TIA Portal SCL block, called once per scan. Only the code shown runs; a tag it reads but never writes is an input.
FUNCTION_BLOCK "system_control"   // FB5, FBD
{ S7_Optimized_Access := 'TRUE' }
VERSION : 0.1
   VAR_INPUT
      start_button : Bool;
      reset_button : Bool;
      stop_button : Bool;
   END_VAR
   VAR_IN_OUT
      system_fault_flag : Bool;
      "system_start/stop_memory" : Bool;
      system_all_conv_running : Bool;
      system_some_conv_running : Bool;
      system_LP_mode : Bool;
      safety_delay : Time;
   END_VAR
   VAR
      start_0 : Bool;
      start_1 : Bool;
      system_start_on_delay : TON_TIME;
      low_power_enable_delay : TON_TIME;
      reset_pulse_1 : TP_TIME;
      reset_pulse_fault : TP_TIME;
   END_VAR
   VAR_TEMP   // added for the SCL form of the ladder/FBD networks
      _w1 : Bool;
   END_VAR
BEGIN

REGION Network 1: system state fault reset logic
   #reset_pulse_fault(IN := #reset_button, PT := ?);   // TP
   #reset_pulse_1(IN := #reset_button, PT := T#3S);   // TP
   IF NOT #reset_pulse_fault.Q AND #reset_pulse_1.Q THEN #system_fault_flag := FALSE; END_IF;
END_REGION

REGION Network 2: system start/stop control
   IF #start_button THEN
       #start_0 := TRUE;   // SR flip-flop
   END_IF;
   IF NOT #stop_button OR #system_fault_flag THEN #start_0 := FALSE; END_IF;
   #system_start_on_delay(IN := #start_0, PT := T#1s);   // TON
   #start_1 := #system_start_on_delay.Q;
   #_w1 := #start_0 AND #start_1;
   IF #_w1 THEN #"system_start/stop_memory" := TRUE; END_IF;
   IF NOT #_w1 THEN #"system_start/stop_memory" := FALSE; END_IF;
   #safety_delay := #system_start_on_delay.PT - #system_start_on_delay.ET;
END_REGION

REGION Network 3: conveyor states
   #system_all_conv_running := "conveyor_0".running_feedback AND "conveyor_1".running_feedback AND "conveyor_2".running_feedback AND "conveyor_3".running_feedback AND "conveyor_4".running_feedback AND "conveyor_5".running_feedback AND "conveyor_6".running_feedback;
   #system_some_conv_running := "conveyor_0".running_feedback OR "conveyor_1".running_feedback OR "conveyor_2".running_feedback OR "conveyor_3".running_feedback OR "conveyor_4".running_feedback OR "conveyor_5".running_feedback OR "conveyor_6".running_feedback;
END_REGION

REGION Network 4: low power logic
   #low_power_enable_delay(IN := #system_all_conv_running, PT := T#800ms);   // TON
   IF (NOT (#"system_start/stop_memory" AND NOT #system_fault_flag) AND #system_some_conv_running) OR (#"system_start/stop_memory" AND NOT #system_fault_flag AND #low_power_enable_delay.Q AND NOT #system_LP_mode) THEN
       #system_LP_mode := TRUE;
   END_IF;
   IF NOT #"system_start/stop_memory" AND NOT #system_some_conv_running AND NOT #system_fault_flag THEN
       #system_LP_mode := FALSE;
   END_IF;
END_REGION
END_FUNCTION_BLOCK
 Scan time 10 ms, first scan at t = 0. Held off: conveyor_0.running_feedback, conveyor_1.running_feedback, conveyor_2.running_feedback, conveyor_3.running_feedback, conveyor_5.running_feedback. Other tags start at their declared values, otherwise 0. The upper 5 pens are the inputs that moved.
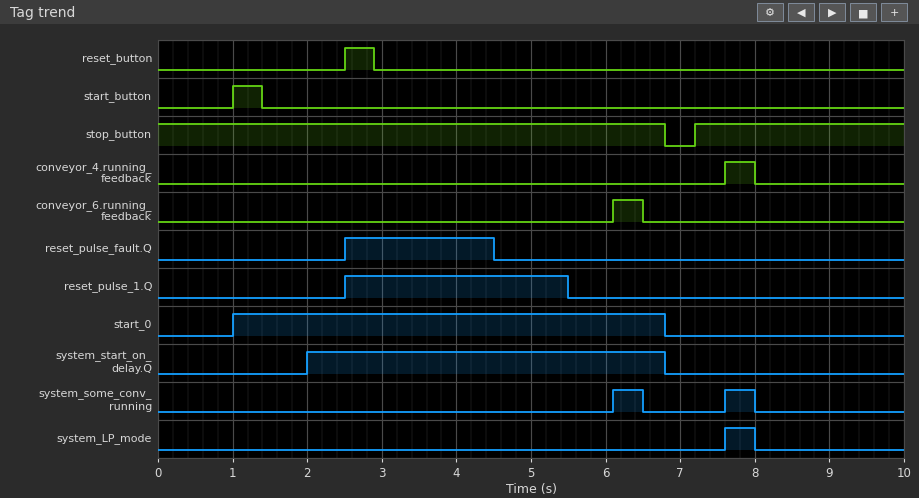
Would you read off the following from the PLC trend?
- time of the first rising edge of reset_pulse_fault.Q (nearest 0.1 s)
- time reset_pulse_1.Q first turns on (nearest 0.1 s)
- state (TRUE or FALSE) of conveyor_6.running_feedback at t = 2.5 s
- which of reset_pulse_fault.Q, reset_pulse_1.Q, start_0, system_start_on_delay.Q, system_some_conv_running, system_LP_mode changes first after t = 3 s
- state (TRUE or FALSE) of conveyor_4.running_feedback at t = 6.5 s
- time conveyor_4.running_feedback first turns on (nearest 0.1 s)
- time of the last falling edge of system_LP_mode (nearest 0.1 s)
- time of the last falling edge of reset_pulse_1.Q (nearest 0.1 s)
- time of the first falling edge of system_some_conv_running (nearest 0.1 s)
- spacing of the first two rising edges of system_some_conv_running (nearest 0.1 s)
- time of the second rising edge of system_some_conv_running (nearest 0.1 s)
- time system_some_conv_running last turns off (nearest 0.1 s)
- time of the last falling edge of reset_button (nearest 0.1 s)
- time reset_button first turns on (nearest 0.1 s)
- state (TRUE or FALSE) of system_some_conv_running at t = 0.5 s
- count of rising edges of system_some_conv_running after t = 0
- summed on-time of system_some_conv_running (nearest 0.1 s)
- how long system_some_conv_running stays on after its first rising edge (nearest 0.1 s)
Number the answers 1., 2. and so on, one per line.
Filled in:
1. 2.5 s
2. 2.5 s
3. FALSE
4. reset_pulse_fault.Q
5. FALSE
6. 7.6 s
7. 8.0 s
8. 5.5 s
9. 6.5 s
10. 1.5 s
11. 7.6 s
12. 8.0 s
13. 2.9 s
14. 2.5 s
15. FALSE
16. 2
17. 0.8 s
18. 0.4 s
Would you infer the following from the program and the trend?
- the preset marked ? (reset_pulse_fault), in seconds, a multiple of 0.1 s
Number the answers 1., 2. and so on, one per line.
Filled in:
1. 2.0 s
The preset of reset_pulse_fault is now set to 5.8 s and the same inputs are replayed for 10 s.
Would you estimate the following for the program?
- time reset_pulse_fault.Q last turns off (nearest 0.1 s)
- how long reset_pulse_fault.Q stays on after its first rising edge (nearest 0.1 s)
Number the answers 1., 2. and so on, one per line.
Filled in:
1. 8.3 s
2. 5.8 s
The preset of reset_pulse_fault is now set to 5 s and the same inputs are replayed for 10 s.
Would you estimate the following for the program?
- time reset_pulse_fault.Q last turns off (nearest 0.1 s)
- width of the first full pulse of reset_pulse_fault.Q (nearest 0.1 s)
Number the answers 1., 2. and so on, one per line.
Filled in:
1. 7.5 s
2. 5.0 s
